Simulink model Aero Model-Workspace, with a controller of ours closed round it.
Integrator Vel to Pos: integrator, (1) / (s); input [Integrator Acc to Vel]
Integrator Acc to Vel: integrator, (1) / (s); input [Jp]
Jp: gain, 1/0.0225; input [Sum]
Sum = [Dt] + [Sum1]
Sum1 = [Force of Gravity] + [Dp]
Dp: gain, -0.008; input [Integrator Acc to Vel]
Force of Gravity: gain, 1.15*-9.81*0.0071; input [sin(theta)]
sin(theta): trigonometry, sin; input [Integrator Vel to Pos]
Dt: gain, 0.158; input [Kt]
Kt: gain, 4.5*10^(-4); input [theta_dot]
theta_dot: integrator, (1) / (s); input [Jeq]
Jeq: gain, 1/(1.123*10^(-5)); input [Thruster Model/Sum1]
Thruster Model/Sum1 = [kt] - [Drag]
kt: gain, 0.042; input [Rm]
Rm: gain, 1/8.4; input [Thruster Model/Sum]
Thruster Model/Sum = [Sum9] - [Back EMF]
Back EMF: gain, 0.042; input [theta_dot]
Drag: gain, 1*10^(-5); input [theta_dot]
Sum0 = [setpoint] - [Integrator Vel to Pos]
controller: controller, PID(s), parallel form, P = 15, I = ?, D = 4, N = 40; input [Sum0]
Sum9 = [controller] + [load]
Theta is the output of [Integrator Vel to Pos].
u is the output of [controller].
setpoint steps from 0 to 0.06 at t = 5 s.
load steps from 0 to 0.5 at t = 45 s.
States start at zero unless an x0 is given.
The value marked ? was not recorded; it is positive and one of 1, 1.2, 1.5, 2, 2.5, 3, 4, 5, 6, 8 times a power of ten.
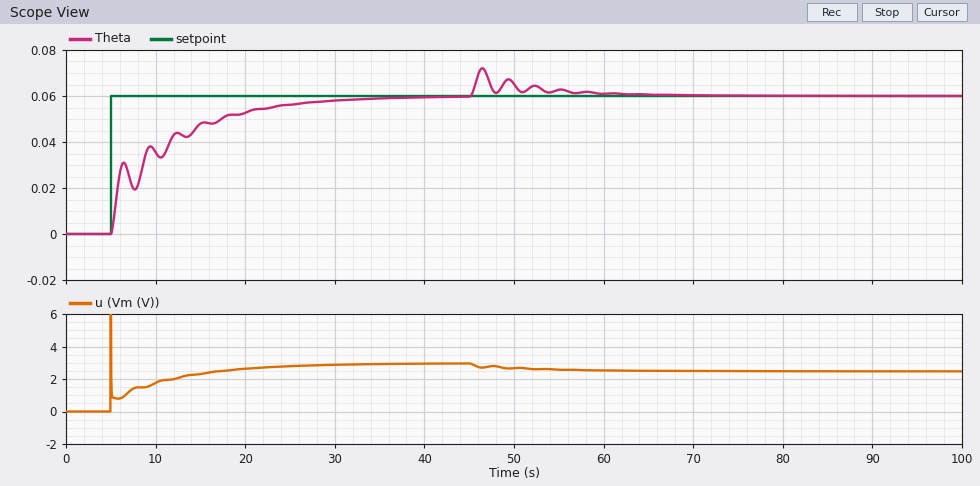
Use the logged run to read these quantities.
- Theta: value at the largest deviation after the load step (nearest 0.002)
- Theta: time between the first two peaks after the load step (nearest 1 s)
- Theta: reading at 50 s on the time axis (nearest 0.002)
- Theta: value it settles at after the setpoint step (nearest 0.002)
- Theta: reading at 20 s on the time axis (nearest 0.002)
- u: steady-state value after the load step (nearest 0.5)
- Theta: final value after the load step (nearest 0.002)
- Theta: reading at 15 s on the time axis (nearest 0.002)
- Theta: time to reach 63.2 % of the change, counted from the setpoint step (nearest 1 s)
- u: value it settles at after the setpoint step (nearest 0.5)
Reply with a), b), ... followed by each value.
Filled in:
a) 0.072
b) 3 s
c) 0.066
d) 0.060
e) 0.052
f) 2.5
g) 0.060
h) 0.048
i) 4 s
j) 3.0
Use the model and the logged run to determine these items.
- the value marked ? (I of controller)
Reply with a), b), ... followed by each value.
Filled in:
a) 8
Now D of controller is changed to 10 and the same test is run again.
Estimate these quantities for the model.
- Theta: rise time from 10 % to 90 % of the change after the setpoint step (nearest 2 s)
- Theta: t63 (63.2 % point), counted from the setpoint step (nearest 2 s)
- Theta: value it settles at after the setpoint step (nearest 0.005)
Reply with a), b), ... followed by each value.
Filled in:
a) 16 s
b) 6 s
c) 0.060
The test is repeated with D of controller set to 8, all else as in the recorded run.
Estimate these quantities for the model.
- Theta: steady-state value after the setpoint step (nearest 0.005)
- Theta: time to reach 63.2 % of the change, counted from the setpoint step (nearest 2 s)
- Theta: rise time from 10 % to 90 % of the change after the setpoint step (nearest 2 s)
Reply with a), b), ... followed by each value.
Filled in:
a) 0.060
b) 6 s
c) 16 s
